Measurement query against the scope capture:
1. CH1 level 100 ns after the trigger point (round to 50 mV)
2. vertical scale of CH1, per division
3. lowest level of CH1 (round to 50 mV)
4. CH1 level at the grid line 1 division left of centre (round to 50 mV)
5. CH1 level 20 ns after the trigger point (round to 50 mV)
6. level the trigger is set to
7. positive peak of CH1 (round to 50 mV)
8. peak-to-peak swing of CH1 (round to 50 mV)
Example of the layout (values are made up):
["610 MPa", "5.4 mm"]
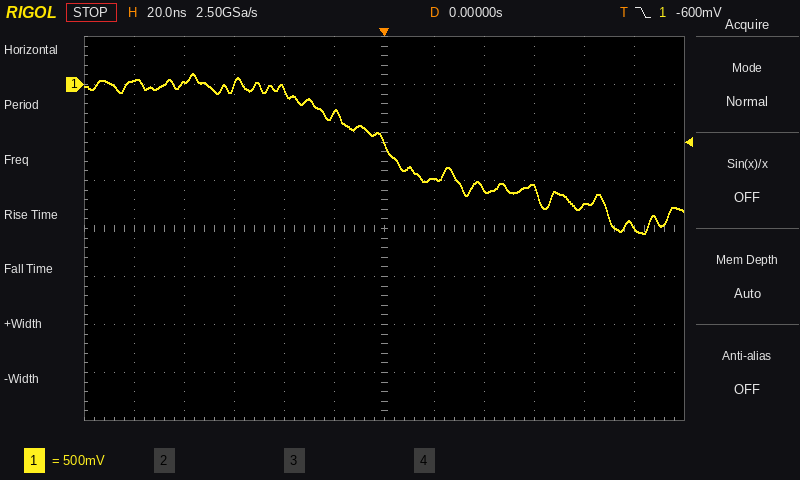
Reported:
["-1.50 V", "500 mV", "-1.55 V", "-300 mV", "-1.00 V", "-600 mV", "100 mV", "1.65 V"]
